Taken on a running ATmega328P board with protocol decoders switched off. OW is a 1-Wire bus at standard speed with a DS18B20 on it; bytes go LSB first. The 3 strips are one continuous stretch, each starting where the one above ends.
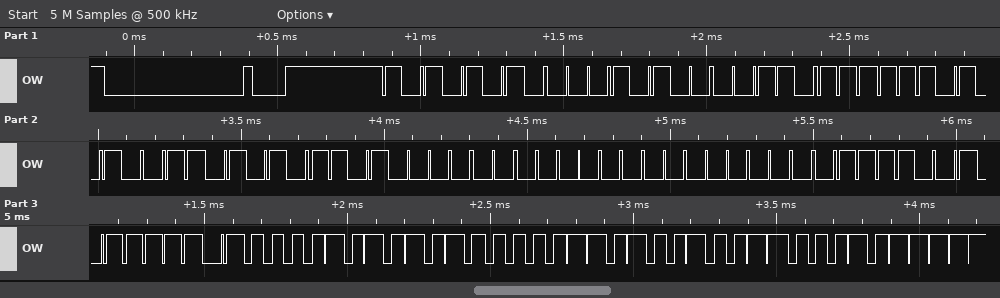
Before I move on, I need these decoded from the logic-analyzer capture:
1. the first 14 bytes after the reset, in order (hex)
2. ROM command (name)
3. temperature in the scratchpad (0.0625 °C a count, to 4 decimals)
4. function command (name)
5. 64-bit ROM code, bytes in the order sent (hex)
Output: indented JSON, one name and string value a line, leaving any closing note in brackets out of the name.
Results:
{
  "the first 14 bytes after the reset, in order": "55 28 EC 57 56 0B 00 00 9E BE 50 05 4B 46",
  "ROM command": "Match ROM",
  "temperature in the scratchpad": "85.0000 °C",
  "function command": "Read Scratchpad",
  "64-bit ROM code, bytes in the order sent": "28 EC 57 56 0B 00 00 9E"
}
